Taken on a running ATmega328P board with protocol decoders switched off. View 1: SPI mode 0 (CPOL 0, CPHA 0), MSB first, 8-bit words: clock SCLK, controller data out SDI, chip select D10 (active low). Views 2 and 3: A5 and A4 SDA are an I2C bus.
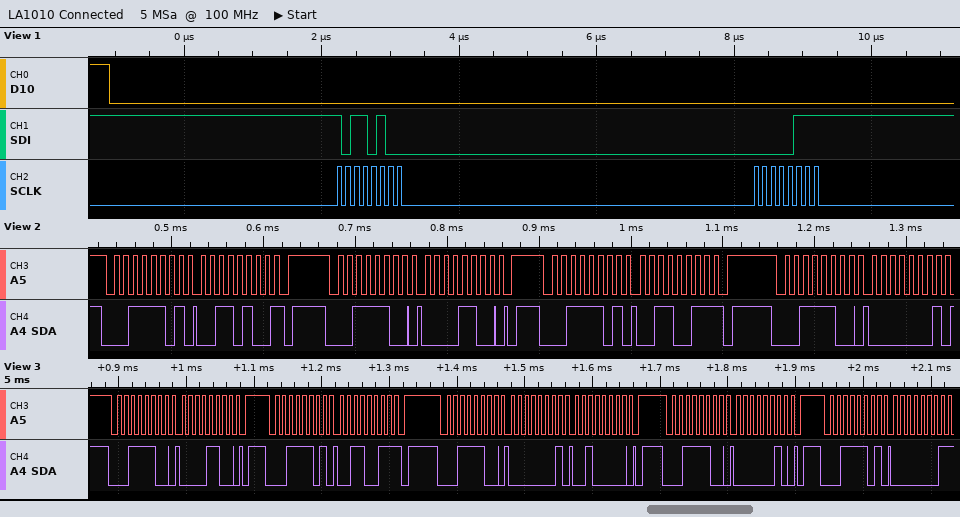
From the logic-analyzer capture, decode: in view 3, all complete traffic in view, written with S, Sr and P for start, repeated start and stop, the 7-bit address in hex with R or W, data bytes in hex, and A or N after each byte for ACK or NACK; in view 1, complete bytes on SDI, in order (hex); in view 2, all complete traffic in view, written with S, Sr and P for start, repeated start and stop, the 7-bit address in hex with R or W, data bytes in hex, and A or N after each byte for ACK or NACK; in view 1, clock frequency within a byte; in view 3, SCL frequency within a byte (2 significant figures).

S 1EW A 0C A P S 1ER A 33 N P S 1EW A 01 A 20 A P S 1EW A 02 A P S 1ER A 01 N
0xB4 0x07
S 1ER A 34 N P S 1EW A 0C A P S 1ER A 33 N P S 1EW A 01 A
8 MHz
100 kHz
